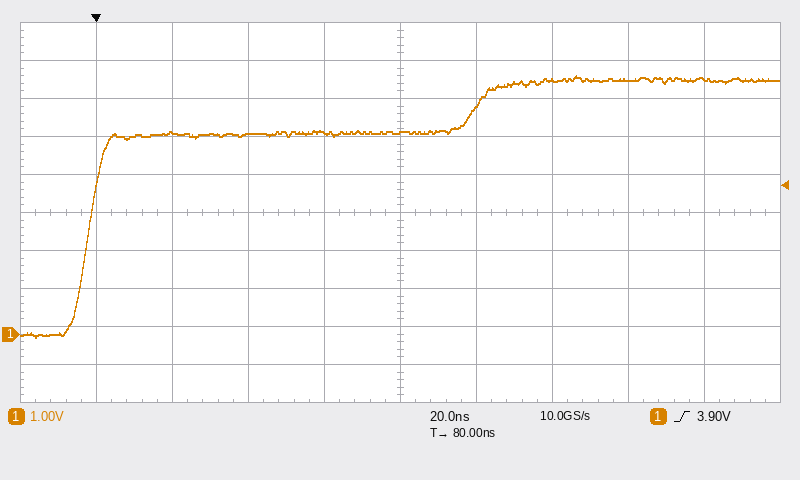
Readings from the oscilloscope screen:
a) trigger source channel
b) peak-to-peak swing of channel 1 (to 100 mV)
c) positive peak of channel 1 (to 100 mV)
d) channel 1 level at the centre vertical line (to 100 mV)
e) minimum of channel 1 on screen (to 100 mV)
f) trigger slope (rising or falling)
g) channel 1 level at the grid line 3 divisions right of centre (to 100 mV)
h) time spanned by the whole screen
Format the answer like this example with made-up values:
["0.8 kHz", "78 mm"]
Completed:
["channel 1", "6.9 V", "6.8 V", "5.3 V", "-100 mV", "rising", "6.7 V", "200 ns"]
